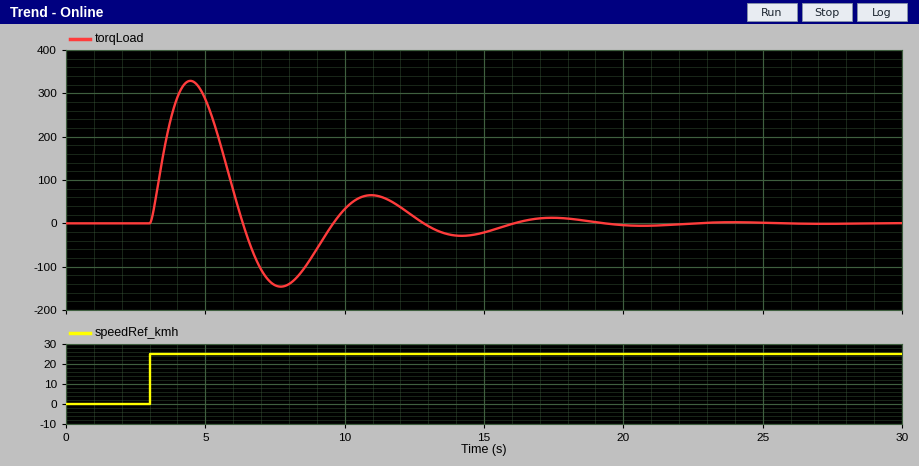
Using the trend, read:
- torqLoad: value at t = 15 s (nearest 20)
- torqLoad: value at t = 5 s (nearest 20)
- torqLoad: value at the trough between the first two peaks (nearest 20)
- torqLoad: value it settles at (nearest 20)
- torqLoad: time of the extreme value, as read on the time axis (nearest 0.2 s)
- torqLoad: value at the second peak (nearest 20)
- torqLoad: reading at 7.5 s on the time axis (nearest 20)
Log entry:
-20
280
-140
0
4.4 s
60
-140
